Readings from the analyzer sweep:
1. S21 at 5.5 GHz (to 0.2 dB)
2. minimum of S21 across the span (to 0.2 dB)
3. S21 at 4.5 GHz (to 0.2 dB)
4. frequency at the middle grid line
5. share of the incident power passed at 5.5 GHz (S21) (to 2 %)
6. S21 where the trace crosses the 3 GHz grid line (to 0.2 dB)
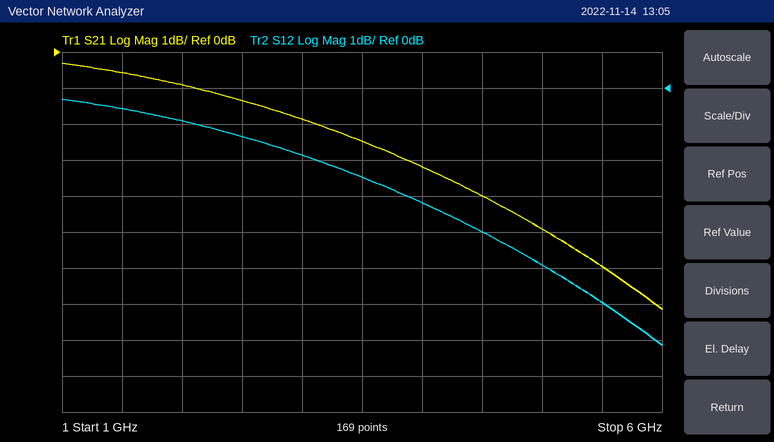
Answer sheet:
-6.0 dB
-7.2 dB
-4.0 dB
3.5 GHz
26 %
-1.8 dB
